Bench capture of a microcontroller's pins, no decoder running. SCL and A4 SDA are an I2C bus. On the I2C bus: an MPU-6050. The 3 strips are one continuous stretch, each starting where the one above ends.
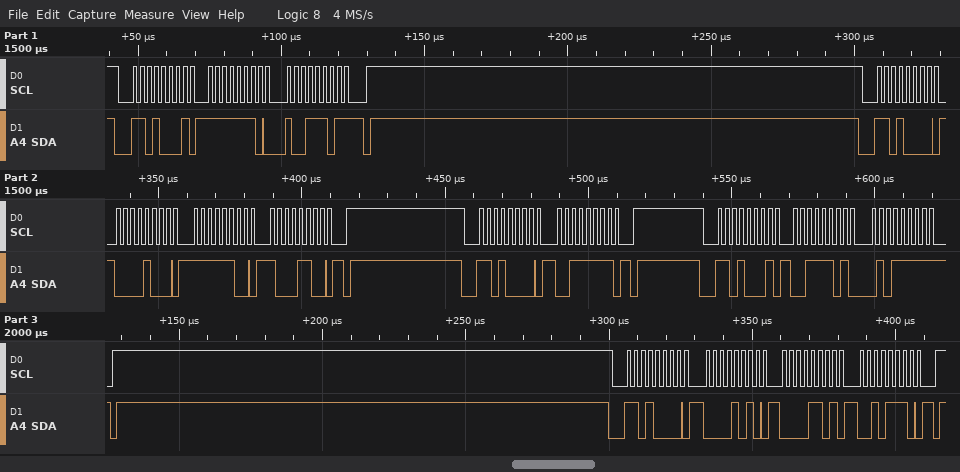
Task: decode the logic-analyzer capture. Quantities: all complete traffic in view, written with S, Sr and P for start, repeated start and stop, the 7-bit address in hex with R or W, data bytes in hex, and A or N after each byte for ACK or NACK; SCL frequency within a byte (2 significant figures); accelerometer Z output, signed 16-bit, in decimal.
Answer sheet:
S 68R A FE A 9D N P S 68W A 08 A FC A 8C A P S 68W A 3F A P S 68R A 3D A 5F N P S 68W A 0A A 0D A 2E A P
400 kHz
15711
